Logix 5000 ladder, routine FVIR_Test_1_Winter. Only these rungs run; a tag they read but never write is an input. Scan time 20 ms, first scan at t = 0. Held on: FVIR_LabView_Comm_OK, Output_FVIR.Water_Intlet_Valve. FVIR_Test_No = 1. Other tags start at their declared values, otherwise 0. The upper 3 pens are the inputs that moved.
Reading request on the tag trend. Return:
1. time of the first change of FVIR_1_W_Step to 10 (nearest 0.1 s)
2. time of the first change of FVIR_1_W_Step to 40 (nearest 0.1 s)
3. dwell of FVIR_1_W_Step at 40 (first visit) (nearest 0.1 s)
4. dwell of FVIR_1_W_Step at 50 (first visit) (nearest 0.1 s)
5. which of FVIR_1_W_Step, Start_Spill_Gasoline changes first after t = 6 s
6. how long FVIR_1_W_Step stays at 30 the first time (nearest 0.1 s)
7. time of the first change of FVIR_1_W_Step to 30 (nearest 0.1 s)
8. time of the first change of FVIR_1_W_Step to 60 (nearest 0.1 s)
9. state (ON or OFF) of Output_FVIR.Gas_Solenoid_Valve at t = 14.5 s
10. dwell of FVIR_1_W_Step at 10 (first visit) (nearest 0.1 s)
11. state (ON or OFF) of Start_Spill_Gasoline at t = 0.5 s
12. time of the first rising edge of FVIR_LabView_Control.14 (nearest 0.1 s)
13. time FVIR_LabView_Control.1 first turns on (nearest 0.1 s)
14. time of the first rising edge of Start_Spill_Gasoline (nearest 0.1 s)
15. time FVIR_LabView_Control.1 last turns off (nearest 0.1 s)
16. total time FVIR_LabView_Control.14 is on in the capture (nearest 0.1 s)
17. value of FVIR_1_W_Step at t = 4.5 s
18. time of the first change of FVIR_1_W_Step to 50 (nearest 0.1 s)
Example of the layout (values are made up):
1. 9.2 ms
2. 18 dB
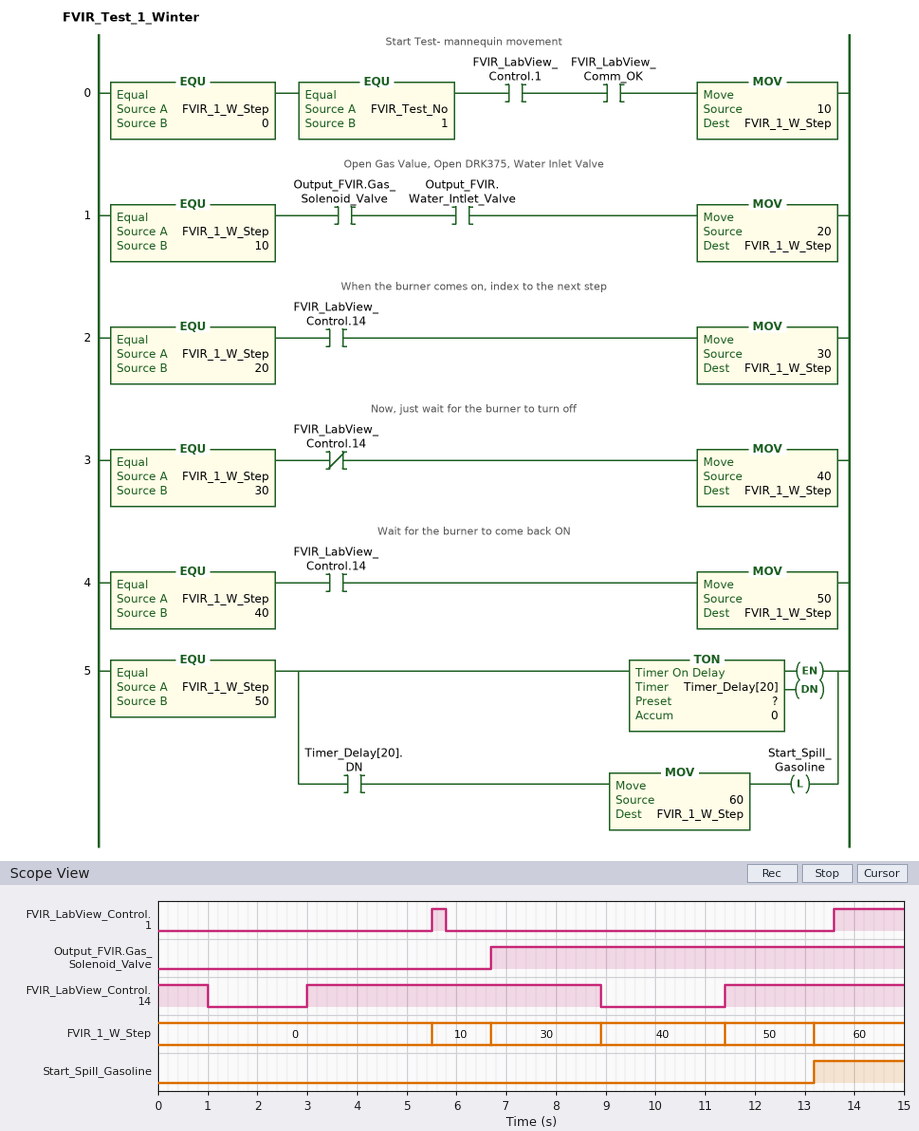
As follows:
1. 5.5 s
2. 8.9 s
3. 2.5 s
4. 1.8 s
5. FVIR_1_W_Step
6. 2.2 s
7. 6.7 s
8. 13.2 s
9. ON
10. 1.2 s
11. OFF
12. 3.0 s
13. 5.5 s
14. 13.2 s
15. 5.8 s
16. 10.5 s
17. 0
18. 11.4 s
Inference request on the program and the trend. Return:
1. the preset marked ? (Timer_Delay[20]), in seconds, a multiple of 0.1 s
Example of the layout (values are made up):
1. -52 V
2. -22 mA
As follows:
1. 1.8 s
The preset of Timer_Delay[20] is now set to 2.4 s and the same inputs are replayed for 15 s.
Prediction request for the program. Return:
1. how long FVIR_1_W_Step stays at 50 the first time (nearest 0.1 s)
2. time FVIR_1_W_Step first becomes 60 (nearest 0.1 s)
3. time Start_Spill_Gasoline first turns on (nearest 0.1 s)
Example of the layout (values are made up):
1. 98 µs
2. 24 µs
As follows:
1. 2.4 s
2. 13.8 s
3. 13.8 s
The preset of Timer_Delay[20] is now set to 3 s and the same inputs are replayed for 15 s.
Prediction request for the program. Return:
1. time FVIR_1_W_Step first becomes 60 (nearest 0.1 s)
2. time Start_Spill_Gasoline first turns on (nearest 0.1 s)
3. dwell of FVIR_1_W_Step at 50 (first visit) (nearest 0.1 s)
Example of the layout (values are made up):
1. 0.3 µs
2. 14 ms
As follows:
1. 14.4 s
2. 14.4 s
3. 3.0 s
